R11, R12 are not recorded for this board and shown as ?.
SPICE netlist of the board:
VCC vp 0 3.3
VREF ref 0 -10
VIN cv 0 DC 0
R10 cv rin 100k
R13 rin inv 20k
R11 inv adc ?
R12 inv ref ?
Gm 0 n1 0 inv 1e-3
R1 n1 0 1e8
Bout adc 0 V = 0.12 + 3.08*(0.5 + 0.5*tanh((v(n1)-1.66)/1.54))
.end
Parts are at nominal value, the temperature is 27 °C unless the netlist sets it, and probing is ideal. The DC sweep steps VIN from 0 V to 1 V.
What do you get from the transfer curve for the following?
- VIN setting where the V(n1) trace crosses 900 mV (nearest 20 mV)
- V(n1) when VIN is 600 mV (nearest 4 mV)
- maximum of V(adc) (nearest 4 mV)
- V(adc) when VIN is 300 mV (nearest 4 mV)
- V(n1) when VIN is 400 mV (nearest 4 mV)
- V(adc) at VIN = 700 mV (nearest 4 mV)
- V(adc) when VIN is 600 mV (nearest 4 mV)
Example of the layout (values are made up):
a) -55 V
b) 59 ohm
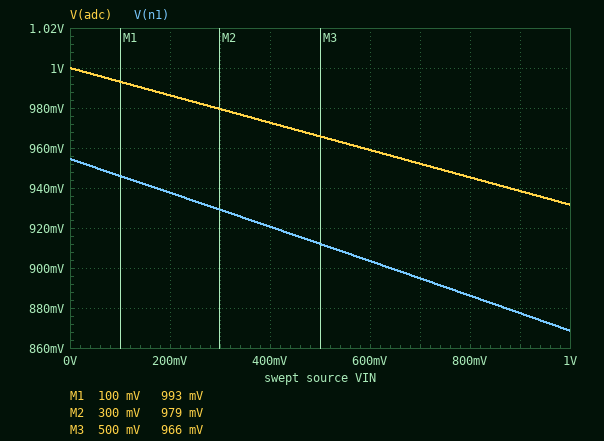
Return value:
a) 640 mV
b) 904 mV
c) 1.000 V
d) 980 mV
e) 920 mV
f) 952 mV
g) 960 mV
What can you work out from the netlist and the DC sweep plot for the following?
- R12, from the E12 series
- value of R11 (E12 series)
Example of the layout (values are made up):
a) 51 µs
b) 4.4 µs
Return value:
a) 82 kΩ
b) 8.2 kΩ
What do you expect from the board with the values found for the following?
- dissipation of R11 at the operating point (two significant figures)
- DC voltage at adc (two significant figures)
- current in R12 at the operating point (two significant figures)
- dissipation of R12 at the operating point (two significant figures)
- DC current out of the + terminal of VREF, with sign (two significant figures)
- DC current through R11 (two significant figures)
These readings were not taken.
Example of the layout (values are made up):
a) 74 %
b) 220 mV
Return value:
a) 120 µW
b) 1.0 V
c) 120 µA
d) 1.2 mW
e) -120 µA
f) 120 µA
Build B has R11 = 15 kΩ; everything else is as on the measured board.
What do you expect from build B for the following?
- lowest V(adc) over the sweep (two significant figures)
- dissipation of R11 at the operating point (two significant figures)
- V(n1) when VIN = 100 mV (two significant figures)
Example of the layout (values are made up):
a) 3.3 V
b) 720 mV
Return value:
a) 1.7 V
b) 220 µW
c) 1.8 V
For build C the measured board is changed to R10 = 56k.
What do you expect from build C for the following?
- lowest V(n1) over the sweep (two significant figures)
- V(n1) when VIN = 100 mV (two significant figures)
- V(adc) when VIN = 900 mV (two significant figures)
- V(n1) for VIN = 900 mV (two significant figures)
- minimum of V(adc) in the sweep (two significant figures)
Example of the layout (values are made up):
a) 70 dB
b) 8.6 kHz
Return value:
a) 820 mV
b) 940 mV
c) 900 mV
d) 830 mV
e) 890 mV
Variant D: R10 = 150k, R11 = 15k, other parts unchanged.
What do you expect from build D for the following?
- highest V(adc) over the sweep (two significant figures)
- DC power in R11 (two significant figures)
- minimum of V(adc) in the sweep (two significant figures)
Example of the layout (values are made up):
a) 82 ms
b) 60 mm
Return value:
a) 1.8 V
b) 220 µW
c) 1.7 V
